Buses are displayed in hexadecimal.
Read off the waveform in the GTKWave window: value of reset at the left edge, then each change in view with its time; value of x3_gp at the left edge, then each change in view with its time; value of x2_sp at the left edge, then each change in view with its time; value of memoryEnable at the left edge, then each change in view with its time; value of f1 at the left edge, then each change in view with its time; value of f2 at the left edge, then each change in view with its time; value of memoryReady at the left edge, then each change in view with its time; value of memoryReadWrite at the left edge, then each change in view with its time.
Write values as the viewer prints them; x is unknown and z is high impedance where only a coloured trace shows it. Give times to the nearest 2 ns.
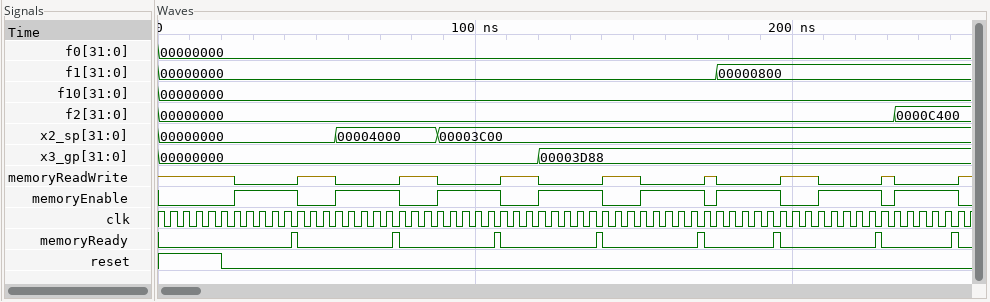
1, 0 at 20 ns
00000000, 00003D88 at 120 ns
00000000, 00004000 at 56 ns, 00003C00 at 88 ns
0, 1 at 24 ns, 0 at 44 ns, 1 at 56 ns, 0 at 76 ns, 1 at 88 ns, 0 at 108 ns, 1 at 120 ns, 0 at 140 ns, 1 at 152 ns, 0 at 172 ns, 1 at 176 ns, 0 at 196 ns, 1 at 208 ns, 0 at 228 ns, 1 at 232 ns, 0 at 252 ns
00000000, 00000800 at 176 ns
00000000, 0000C400 at 232 ns
0, 1 at 42 ns, 0 at 44 ns, 1 at 74 ns, 0 at 76 ns, 1 at 106 ns, 0 at 108 ns, 1 at 138 ns, 0 at 140 ns, 1 at 170 ns, 0 at 172 ns, 1 at 194 ns, 0 at 196 ns, 1 at 226 ns, 0 at 228 ns, 1 at 250 ns, 0 at 252 ns
z, 0 at 24 ns, z at 44 ns, 0 at 56 ns, z at 76 ns, 0 at 88 ns, z at 108 ns, 0 at 120 ns, z at 140 ns, 0 at 152 ns, z at 172 ns, 0 at 176 ns, z at 196 ns, 0 at 208 ns, z at 228 ns, 0 at 232 ns, z at 252 ns
